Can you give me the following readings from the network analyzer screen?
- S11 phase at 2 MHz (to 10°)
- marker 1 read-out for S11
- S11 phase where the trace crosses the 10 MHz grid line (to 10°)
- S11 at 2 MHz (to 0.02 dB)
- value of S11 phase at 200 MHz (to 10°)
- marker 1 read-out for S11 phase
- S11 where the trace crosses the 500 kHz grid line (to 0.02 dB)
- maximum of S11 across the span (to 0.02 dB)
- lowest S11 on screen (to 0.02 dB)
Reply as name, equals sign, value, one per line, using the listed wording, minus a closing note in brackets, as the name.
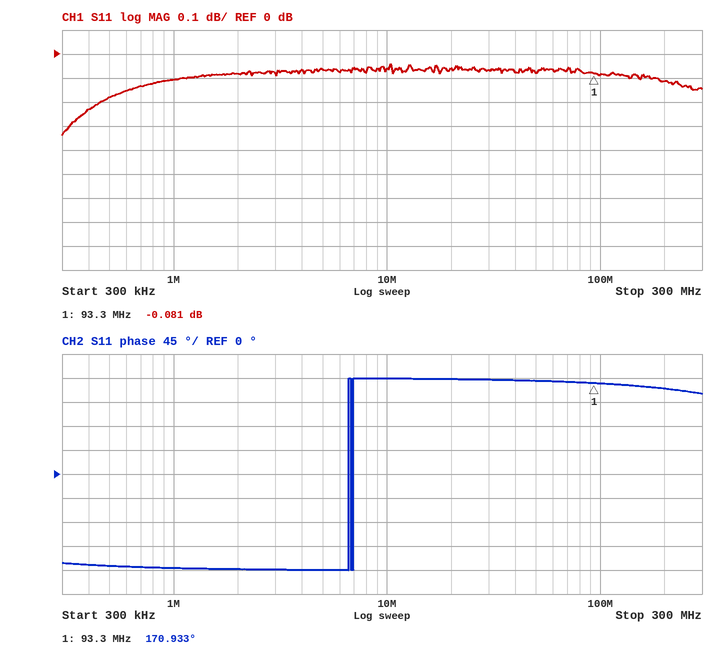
S11 phase at 2 MHz = -180°
marker 1 read-out for S11 = -0.081 dB
S11 phase where the trace crosses the 10 MHz grid line = 180°
S11 at 2 MHz = -0.08 dB
value of S11 phase at 200 MHz = 160°
marker 1 read-out for S11 phase = 170.933°
S11 where the trace crosses the 500 kHz grid line = -0.18 dB
maximum of S11 across the span = -0.04 dB
lowest S11 on screen = -0.34 dB
